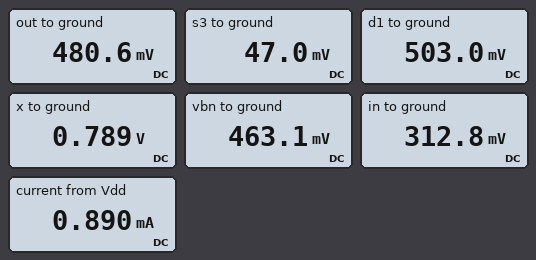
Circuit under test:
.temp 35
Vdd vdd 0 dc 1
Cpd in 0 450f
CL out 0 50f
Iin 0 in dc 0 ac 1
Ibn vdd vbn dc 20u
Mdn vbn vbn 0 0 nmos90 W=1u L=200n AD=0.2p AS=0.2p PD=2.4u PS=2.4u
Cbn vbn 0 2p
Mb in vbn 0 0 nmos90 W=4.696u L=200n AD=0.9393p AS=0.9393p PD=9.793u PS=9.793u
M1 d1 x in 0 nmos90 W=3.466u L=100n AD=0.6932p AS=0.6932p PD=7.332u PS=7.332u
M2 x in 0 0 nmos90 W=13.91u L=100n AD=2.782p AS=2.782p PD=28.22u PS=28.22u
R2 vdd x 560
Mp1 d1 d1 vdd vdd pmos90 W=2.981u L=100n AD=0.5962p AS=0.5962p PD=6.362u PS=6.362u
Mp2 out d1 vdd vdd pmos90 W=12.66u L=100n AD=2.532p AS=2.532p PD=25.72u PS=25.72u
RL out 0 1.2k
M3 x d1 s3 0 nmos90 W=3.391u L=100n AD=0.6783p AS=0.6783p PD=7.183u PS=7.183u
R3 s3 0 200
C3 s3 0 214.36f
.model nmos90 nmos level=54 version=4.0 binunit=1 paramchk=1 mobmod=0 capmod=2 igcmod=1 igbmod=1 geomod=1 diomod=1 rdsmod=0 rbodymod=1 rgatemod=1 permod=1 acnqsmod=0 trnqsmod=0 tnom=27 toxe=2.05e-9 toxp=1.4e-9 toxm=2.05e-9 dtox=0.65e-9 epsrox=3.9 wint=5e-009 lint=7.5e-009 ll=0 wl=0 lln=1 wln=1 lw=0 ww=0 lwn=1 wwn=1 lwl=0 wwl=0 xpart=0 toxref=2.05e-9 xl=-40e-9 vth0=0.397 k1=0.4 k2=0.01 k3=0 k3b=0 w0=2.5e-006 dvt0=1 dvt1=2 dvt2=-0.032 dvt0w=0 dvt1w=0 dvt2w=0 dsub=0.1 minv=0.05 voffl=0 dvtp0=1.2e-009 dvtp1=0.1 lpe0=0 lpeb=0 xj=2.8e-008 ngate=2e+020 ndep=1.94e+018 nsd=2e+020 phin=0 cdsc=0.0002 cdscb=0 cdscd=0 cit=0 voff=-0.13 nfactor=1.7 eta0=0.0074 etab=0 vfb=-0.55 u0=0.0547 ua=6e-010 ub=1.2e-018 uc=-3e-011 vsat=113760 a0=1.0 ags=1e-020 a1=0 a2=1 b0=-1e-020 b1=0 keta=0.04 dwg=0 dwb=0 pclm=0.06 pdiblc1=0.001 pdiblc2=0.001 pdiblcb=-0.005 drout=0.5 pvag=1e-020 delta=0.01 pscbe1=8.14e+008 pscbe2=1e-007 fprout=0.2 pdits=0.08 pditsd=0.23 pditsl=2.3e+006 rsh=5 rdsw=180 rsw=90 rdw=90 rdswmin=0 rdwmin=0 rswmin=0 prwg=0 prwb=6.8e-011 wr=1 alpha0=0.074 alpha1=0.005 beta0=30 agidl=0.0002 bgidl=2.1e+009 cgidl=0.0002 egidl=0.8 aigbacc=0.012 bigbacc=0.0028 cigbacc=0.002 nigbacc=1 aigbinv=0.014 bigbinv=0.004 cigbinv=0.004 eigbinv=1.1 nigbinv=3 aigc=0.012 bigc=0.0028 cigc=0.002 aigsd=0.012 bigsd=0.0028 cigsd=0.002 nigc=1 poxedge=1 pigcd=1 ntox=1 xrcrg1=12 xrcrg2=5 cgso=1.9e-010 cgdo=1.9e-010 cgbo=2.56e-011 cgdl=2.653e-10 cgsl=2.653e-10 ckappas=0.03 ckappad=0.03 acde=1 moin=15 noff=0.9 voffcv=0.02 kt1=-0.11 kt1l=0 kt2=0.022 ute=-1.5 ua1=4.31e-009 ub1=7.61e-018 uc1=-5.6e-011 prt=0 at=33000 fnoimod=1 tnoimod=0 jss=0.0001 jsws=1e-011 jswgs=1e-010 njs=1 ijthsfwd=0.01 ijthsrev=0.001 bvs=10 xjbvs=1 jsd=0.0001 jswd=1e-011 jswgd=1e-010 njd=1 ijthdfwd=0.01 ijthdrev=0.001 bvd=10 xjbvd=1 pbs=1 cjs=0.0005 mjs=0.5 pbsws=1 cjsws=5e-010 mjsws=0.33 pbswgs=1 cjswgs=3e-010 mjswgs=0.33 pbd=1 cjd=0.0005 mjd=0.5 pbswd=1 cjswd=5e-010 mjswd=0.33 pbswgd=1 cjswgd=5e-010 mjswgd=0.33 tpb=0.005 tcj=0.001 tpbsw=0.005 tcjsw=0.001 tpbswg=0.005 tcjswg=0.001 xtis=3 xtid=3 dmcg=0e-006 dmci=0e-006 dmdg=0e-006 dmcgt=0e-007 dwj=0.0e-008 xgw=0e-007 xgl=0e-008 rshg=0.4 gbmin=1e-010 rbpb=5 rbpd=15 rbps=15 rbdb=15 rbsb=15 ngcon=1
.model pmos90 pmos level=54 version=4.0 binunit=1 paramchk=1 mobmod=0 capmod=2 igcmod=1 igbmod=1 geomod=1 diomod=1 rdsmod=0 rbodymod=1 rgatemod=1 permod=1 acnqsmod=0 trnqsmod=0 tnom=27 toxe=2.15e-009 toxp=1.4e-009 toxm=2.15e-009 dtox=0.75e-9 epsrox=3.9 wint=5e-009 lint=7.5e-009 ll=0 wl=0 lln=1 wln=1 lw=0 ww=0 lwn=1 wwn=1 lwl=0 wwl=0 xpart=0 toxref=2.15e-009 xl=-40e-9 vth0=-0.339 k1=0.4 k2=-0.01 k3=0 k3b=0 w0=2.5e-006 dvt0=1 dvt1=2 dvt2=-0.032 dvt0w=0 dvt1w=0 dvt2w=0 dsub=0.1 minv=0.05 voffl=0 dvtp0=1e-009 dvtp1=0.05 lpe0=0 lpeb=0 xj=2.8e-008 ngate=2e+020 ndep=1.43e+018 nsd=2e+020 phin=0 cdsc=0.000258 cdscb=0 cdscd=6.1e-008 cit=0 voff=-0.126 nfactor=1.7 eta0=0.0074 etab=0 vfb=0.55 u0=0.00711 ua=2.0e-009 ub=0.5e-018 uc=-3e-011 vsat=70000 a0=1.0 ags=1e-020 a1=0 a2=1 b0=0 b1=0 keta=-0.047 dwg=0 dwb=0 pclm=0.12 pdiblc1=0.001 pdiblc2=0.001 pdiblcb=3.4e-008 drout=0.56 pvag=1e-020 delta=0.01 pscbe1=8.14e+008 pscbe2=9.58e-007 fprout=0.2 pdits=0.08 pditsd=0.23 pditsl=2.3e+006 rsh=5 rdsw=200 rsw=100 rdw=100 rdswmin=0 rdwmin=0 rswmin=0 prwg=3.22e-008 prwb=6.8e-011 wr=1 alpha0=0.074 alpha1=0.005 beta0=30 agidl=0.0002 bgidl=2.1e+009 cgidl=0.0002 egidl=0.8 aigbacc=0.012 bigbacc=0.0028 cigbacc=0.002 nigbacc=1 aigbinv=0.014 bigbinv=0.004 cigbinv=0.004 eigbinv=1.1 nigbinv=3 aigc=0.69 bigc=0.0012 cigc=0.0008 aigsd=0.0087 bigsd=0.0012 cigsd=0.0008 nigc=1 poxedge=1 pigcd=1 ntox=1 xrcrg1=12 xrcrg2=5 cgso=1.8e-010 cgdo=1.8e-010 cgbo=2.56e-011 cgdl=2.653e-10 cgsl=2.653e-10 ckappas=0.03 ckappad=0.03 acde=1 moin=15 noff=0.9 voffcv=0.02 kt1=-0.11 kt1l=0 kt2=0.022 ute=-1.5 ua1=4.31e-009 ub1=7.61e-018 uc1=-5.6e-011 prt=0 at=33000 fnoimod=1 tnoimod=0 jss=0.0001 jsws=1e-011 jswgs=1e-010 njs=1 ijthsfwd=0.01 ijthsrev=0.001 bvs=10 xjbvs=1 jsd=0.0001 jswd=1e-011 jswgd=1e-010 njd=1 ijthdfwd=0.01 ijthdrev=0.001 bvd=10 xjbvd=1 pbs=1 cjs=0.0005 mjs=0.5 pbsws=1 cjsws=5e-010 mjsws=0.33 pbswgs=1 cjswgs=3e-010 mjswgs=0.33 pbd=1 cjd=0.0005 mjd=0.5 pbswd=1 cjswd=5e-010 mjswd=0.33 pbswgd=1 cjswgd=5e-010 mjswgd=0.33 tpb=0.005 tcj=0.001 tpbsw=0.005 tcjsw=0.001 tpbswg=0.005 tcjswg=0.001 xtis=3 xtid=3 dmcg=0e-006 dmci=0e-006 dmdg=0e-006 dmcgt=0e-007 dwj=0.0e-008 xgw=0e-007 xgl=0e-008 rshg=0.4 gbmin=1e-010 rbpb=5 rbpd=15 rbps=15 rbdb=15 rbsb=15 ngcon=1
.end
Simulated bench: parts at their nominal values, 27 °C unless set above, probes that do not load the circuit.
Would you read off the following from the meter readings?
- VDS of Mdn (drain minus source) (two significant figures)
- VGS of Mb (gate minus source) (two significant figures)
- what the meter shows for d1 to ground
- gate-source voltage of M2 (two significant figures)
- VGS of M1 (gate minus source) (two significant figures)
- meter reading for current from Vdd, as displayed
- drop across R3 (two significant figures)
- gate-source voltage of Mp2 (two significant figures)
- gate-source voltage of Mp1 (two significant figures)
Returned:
460 mV
460 mV
503.0 mV
310 mV
480 mV
0.890 mA
47 mV
-500 mV
-500 mV
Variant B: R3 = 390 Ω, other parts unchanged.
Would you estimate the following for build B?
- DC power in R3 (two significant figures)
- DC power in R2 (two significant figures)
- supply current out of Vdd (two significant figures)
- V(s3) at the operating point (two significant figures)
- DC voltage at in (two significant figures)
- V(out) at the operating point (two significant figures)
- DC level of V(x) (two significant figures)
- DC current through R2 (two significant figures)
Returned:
12 µW
69 µW
860 µA
68 mV
320 mV
480 mV
800 mV
350 µA
